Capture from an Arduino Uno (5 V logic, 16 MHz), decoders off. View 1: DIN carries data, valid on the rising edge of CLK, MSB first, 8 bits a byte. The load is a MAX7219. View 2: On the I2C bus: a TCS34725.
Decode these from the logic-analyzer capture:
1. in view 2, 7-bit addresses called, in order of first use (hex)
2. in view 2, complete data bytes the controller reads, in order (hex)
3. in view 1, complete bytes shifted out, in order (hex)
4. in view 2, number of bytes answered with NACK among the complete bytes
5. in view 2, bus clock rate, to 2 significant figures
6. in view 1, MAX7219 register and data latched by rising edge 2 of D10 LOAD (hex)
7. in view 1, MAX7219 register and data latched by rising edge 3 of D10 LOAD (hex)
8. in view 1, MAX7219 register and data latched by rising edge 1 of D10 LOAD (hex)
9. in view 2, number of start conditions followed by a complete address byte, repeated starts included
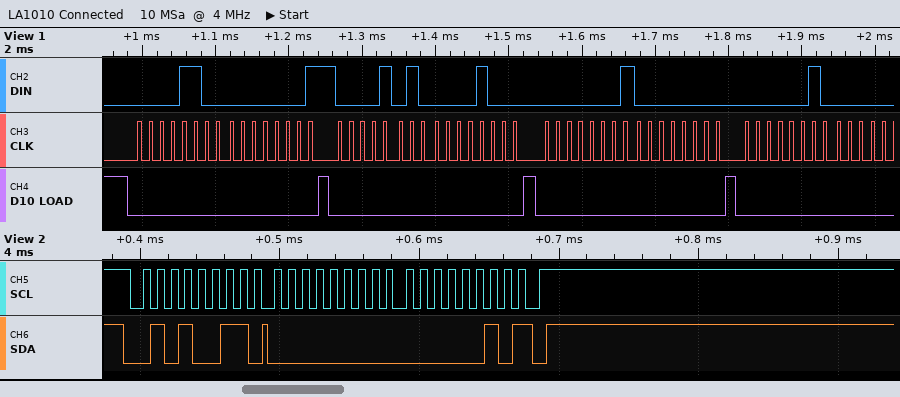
0x29
00 02
0x0C 0x01 0x0A 0x08 0x01 0x00 0x02
1
100 kHz
register 0xA, data 0x08
register 0x1, data 0x00
register 0xC, data 0x01
1
